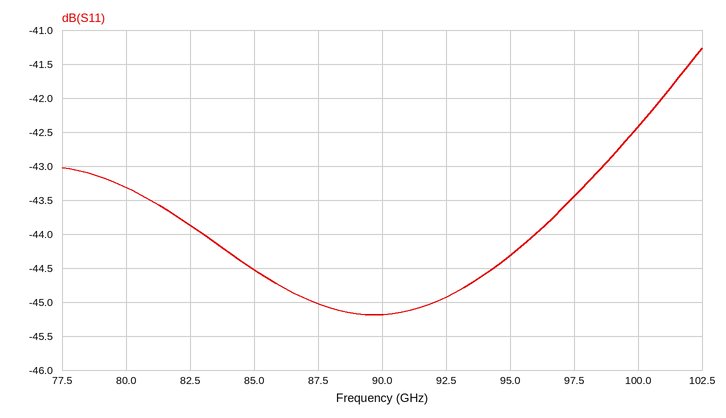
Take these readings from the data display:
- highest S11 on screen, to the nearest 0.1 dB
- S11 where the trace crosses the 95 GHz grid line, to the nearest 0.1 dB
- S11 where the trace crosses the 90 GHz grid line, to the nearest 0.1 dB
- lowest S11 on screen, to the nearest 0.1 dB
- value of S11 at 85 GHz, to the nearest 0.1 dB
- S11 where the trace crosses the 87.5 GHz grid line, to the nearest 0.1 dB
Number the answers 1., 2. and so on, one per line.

1. -41.3 dB
2. -44.3 dB
3. -45.2 dB
4. -45.2 dB
5. -44.5 dB
6. -45.0 dB
